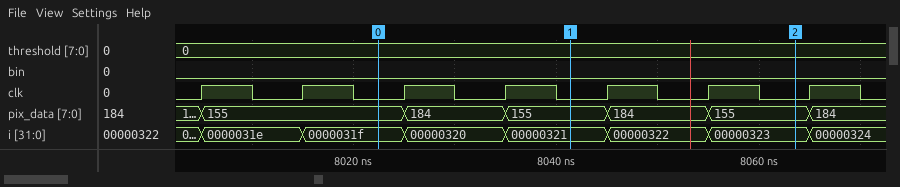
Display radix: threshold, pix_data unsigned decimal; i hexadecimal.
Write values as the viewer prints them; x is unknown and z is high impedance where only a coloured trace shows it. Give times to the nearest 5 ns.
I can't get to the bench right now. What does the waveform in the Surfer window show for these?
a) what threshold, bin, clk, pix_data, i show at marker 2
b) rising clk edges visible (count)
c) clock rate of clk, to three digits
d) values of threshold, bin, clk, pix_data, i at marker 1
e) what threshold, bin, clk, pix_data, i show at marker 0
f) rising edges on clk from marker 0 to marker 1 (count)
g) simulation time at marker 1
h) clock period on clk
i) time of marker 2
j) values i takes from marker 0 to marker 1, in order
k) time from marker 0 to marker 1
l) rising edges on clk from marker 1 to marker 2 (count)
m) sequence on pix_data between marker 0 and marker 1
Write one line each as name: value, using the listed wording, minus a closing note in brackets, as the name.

what threshold, bin, clk, pix_data, i show at marker 2: threshold=0, bin=0, clk=0, pix_data=155, i=00000323
rising clk edges visible: 7
clock rate of clk, to three digits: 100 MHz
values of threshold, bin, clk, pix_data, i at marker 1: threshold=0, bin=0, clk=0, pix_data=155, i=00000321
what threshold, bin, clk, pix_data, i show at marker 0: threshold=0, bin=0, clk=0, pix_data=155, i=0000031f
rising edges on clk from marker 0 to marker 1: 2
simulation time at marker 1: 8040 ns
clock period on clk: 10 ns
time of marker 2: 8065 ns
values i takes from marker 0 to marker 1, in order: 0000031f, 00000320, 00000321
time from marker 0 to marker 1: 20 ns
rising edges on clk from marker 1 to marker 2: 2
sequence on pix_data between marker 0 and marker 1: 155, 184, 155
